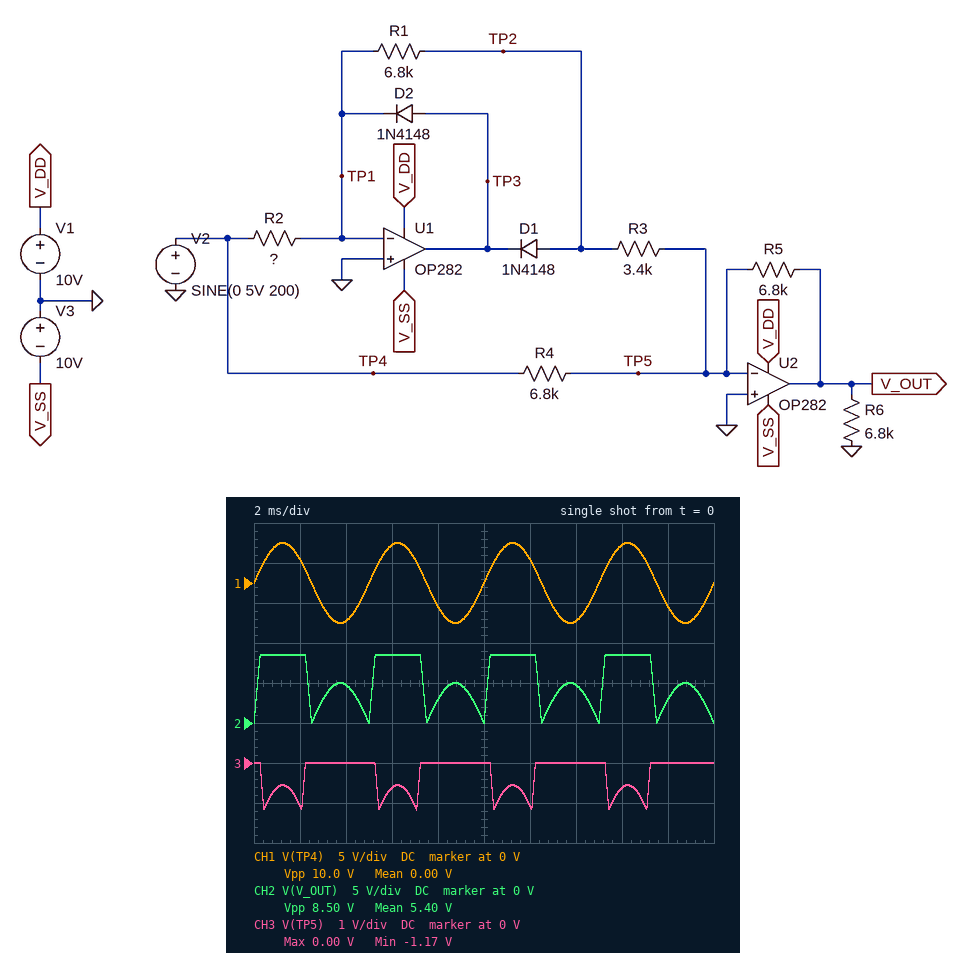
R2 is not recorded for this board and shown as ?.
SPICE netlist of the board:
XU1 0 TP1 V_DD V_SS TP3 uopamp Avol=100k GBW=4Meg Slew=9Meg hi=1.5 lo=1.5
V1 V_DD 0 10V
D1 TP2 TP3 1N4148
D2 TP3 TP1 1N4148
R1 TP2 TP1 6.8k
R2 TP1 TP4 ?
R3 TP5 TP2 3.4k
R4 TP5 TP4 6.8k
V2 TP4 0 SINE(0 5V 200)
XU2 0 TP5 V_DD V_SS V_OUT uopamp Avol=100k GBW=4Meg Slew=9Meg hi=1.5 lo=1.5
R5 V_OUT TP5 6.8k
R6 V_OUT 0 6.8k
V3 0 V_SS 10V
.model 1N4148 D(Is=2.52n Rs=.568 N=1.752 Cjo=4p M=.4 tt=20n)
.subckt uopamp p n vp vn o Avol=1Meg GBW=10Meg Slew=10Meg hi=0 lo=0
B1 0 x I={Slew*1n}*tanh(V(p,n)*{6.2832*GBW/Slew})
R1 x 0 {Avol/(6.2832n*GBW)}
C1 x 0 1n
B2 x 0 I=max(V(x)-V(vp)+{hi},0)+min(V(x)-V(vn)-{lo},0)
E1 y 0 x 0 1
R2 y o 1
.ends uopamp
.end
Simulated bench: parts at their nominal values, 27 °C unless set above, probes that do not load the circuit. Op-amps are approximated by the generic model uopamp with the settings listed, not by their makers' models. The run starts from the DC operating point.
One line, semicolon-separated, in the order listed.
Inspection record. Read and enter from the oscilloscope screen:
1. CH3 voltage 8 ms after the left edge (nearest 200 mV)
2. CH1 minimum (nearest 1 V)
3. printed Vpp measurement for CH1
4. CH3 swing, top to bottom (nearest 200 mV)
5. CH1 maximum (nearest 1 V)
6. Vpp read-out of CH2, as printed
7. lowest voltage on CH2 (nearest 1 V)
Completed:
0 V; -5 V; 10.0 V; 1.2 V; 5 V; 8.50 V; 0 V
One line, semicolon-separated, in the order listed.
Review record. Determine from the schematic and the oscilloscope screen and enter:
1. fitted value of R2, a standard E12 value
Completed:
2.2 kΩ
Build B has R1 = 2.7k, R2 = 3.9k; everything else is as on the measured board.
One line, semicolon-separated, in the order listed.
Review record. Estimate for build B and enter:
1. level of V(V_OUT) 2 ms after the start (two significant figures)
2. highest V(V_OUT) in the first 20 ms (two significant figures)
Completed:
1.1 V; 5.0 V
